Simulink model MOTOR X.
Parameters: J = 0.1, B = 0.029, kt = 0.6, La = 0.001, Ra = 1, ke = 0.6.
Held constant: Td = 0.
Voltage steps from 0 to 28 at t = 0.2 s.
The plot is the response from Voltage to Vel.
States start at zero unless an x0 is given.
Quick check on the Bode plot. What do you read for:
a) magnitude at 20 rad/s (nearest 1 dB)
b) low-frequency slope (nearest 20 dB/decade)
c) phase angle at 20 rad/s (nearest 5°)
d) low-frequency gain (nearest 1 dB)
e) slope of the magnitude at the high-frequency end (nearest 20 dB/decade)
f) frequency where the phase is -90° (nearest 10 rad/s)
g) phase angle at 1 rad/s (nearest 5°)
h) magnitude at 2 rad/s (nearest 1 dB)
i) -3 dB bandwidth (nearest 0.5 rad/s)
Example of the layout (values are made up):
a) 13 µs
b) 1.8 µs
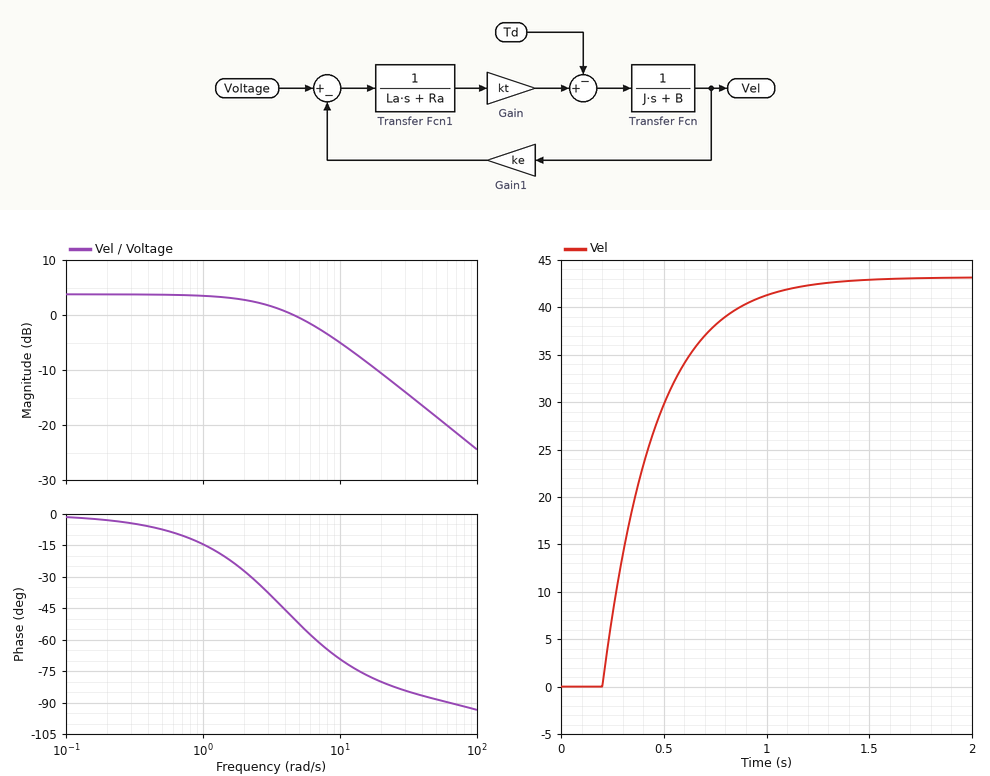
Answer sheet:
a) -11 dB
b) 0 dB/decade
c) -80°
d) 4 dB
e) -20 dB/decade
f) 60 rad/s
g) -15°
h) 3 dB
i) 4.0 rad/s
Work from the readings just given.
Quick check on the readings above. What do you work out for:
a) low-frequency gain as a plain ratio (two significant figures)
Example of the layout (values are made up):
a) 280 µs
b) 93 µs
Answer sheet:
a) 1.6
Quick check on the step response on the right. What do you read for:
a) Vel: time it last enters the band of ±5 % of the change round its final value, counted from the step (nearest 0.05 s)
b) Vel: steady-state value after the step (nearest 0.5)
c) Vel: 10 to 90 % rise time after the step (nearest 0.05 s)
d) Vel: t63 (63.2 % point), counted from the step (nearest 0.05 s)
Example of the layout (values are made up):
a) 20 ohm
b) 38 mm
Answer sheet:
a) 0.75 s
b) 43.0
c) 0.55 s
d) 0.25 s
